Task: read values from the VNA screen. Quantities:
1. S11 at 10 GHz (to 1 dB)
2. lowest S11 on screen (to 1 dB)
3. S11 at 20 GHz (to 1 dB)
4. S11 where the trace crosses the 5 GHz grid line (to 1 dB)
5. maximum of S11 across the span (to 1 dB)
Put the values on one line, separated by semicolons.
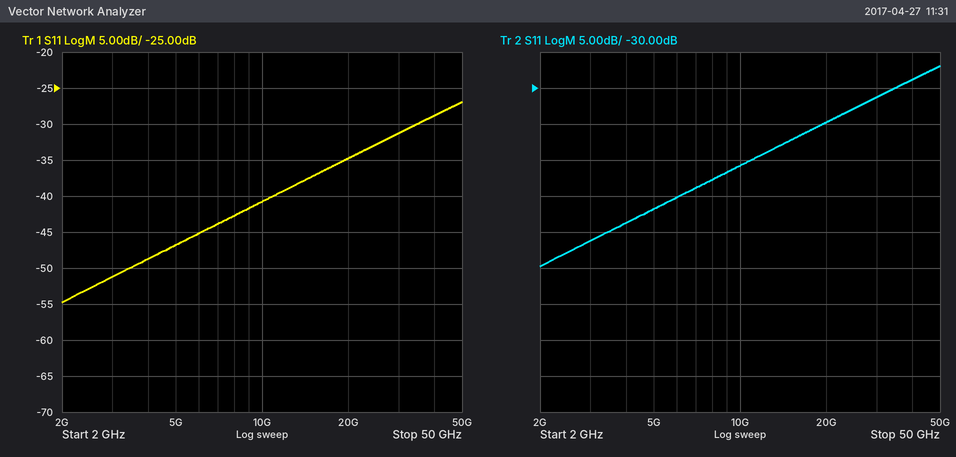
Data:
-41 dB; -55 dB; -35 dB; -47 dB; -27 dB
